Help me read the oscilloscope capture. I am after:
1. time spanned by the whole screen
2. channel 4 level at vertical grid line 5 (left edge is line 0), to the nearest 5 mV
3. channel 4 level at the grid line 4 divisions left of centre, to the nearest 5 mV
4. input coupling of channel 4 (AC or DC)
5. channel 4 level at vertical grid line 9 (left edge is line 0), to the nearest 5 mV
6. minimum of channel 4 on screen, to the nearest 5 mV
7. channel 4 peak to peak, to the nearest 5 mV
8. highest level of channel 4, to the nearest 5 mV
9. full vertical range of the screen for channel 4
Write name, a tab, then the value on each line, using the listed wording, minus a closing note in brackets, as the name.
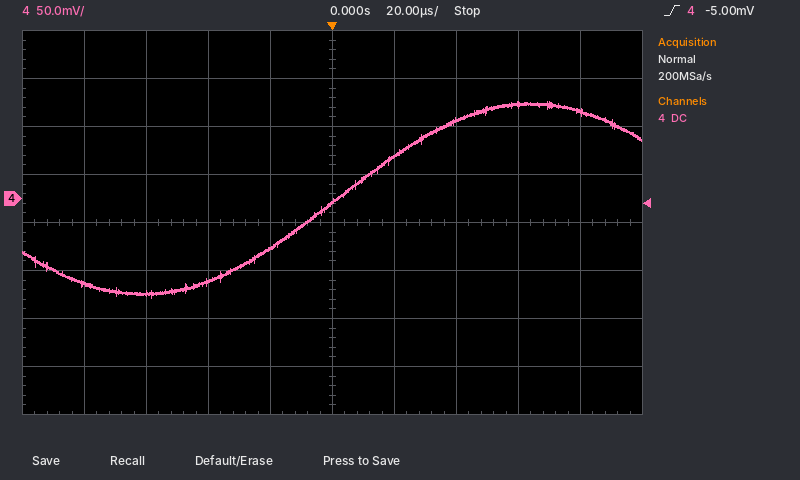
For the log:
time spanned by the whole screen	200 µs
channel 4 level at vertical grid line 5 (left edge is line 0), to the nearest 5 mV	-5 mV
channel 4 level at the grid line 4 divisions left of centre, to the nearest 5 mV	-90 mV
input coupling of channel 4	DC
channel 4 level at vertical grid line 9 (left edge is line 0), to the nearest 5 mV	90 mV
minimum of channel 4 on screen, to the nearest 5 mV	-105 mV
channel 4 peak to peak, to the nearest 5 mV	205 mV
highest level of channel 4, to the nearest 5 mV	100 mV
full vertical range of the screen for channel 4	400 mV
